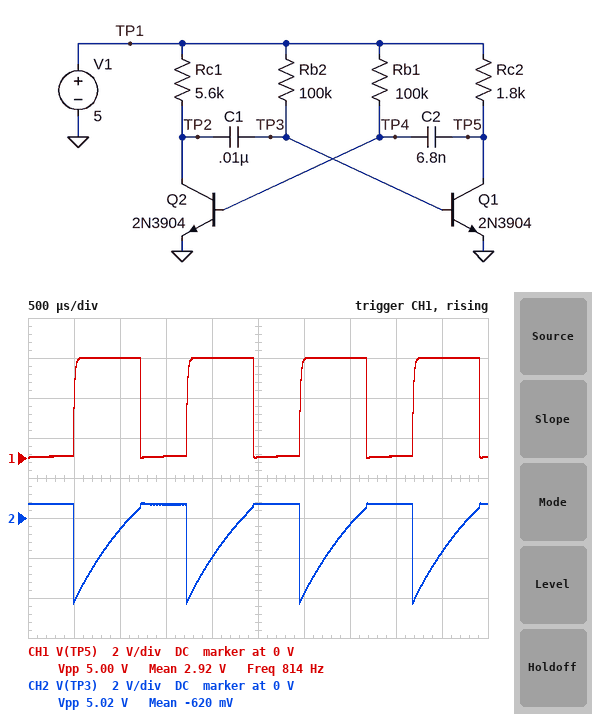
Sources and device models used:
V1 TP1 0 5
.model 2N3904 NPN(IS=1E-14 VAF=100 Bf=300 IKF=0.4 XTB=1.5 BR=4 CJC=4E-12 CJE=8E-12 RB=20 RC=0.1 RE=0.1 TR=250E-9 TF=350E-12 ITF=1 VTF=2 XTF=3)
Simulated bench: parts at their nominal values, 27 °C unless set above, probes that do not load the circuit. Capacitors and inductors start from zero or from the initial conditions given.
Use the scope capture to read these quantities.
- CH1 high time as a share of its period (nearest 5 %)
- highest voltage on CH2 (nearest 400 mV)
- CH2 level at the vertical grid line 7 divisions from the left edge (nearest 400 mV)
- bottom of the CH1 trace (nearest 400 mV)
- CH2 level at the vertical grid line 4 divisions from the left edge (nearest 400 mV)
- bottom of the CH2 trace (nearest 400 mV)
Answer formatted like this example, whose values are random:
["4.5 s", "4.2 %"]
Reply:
["60 %", "800 mV", "-400 mV", "0 V", "-2.0 V", "-4.4 V"]
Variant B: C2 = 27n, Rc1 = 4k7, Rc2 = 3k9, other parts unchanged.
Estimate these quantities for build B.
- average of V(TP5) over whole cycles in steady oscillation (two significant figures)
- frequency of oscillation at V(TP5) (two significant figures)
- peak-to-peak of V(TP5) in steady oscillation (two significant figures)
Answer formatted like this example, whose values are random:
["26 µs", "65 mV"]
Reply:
["1.2 V", "370 Hz", "5.0 V"]
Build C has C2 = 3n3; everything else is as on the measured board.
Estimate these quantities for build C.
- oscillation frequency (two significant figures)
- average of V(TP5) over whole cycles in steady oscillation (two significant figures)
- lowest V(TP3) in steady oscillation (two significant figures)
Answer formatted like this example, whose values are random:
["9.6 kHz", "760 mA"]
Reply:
["1.0 kHz", "3.7 V", "-4.2 V"]
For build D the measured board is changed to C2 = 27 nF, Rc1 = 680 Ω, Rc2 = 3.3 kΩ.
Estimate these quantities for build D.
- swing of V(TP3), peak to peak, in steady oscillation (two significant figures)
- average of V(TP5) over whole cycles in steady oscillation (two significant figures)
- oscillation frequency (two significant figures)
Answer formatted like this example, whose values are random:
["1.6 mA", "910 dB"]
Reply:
["5.1 V", "1.2 V", "370 Hz"]
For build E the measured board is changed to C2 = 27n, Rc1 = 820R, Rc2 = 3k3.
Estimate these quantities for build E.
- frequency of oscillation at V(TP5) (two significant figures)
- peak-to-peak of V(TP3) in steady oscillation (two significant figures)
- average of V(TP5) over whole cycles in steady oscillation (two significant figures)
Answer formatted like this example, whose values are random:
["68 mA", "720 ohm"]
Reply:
["370 Hz", "5.1 V", "1.2 V"]
